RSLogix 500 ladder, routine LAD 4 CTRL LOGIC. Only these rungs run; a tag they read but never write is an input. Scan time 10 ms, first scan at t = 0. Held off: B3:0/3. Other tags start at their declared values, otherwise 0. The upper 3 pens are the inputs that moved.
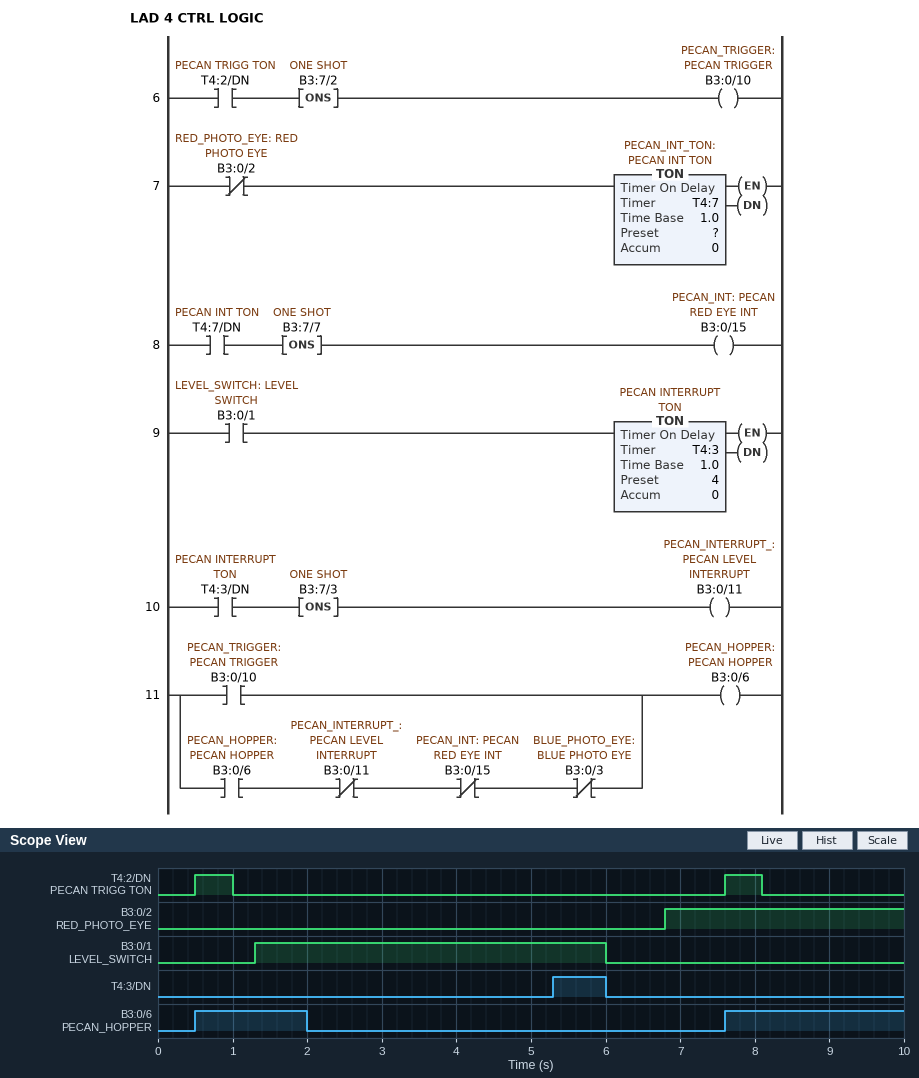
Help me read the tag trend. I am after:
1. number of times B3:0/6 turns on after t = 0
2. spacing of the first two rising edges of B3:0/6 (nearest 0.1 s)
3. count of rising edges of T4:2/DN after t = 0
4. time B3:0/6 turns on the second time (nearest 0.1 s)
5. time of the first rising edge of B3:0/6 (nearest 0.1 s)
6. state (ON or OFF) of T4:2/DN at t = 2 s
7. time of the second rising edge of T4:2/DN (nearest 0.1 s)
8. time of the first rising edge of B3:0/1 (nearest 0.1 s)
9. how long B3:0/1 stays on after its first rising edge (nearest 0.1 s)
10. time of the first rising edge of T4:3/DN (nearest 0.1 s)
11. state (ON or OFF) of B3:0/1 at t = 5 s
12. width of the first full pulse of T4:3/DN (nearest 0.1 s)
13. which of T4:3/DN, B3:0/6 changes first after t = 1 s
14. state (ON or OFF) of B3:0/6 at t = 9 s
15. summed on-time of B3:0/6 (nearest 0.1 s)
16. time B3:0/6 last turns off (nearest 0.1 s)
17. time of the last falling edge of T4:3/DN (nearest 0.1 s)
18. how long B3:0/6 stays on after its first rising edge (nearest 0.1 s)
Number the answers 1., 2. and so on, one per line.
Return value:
1. 2
2. 7.1 s
3. 2
4. 7.6 s
5. 0.5 s
6. OFF
7. 7.6 s
8. 1.3 s
9. 4.7 s
10. 5.3 s
11. ON
12. 0.7 s
13. B3:0/6
14. ON
15. 3.9 s
16. 2.0 s
17. 6.0 s
18. 1.5 s
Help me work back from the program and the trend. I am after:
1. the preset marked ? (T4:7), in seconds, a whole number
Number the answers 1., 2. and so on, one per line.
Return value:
1. 2 s
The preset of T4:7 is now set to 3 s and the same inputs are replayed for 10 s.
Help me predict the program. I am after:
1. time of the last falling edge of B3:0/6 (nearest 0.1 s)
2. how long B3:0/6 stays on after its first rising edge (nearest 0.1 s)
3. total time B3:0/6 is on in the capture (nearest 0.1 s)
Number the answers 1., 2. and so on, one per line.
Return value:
1. 3.0 s
2. 2.5 s
3. 4.9 s
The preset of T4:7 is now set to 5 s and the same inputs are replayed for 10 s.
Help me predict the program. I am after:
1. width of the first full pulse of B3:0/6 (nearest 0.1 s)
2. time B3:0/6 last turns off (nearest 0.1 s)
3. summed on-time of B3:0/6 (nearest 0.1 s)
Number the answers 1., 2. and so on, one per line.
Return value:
1. 4.5 s
2. 5.0 s
3. 6.9 s
